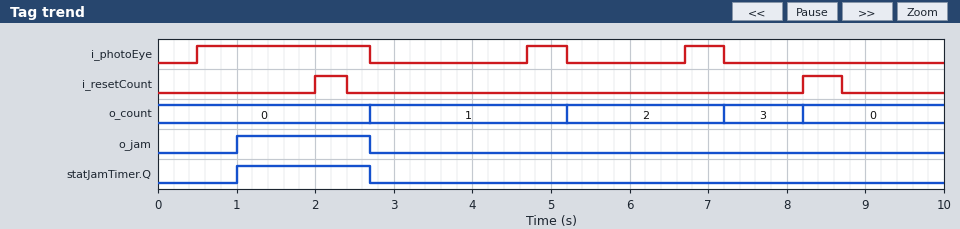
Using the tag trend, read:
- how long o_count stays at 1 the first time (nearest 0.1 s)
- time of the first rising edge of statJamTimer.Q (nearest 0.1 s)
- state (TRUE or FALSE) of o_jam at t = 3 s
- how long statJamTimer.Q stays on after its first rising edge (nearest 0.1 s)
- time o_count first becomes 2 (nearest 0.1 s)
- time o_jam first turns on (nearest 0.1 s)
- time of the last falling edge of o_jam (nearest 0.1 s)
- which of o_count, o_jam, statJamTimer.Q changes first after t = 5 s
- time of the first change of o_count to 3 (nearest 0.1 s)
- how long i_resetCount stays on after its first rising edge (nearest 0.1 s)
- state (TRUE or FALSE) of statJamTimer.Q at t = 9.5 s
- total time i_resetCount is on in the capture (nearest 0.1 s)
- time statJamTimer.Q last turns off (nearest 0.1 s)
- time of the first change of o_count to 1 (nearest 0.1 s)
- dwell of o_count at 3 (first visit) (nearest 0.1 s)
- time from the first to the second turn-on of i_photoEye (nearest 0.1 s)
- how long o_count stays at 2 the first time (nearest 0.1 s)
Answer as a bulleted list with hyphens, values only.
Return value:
- 2.5 s
- 1.0 s
- FALSE
- 1.7 s
- 5.2 s
- 1.0 s
- 2.7 s
- o_count
- 7.2 s
- 0.4 s
- FALSE
- 0.9 s
- 2.7 s
- 2.7 s
- 1.0 s
- 4.2 s
- 2.0 s
